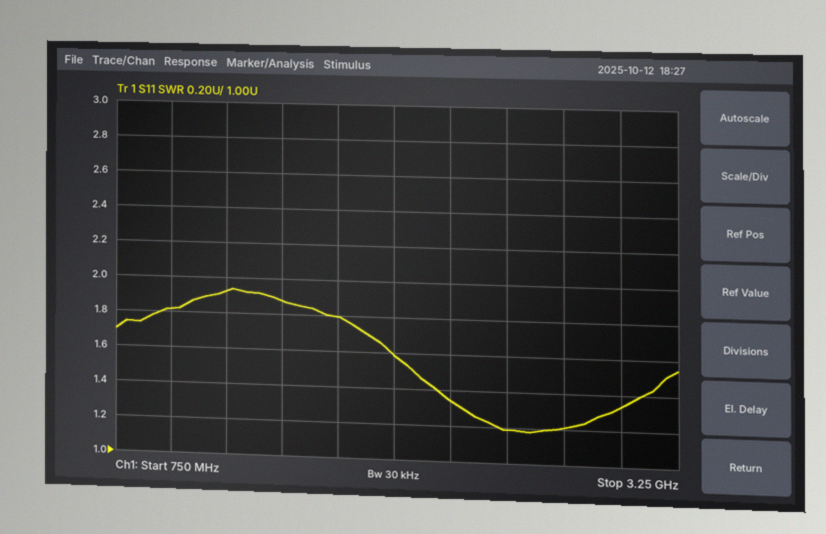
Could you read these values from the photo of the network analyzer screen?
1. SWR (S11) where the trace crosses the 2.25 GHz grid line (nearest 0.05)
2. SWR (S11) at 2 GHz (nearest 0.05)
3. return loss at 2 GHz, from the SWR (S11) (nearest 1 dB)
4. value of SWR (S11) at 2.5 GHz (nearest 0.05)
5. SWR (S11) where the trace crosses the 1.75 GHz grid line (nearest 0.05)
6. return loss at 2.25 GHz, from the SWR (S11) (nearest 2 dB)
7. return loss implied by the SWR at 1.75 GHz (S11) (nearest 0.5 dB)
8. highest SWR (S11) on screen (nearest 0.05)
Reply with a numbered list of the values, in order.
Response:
1. 1.35
2. 1.60
3. 13 dB
4. 1.20
5. 1.80
6. 16 dB
7. 11.0 dB
8. 1.95
